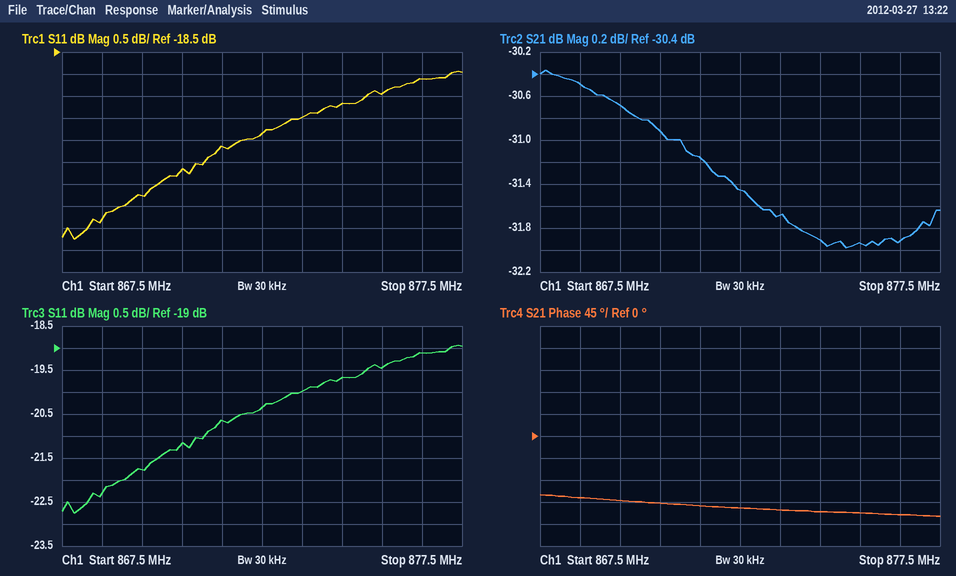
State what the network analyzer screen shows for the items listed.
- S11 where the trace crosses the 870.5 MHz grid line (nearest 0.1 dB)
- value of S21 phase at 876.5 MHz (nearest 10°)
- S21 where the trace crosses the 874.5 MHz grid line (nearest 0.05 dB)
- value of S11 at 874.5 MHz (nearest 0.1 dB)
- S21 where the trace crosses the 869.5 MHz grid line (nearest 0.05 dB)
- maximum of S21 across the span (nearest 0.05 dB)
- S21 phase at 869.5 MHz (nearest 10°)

-21.2 dB
-160°
-31.90 dB
-19.7 dB
-30.70 dB
-30.35 dB
-130°
